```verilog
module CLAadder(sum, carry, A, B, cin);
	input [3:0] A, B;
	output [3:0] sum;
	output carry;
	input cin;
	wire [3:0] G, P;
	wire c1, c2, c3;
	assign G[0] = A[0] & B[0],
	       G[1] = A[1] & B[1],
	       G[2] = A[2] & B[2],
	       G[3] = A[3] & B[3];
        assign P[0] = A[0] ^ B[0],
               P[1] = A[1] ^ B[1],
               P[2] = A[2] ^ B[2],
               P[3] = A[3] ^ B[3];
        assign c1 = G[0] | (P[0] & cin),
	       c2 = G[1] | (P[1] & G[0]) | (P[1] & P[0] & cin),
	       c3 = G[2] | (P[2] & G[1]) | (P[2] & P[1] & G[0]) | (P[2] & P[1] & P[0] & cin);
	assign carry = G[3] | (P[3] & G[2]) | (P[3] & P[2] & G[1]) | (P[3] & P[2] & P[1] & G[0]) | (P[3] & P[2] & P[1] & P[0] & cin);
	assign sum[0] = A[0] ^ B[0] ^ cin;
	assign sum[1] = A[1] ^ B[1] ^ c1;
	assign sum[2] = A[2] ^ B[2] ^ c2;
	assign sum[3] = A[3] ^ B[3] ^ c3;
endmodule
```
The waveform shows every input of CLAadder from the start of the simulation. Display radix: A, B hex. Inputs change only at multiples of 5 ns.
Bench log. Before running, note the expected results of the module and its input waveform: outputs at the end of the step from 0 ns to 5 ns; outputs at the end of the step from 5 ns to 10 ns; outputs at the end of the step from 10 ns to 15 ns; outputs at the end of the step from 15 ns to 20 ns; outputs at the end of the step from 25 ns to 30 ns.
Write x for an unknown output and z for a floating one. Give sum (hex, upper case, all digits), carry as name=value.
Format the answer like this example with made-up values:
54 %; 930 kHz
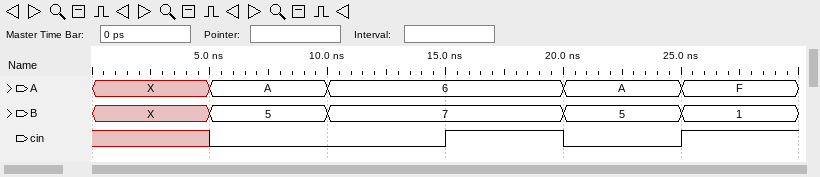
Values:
sum=x, carry=x; sum=F, carry=0; sum=D, carry=0; sum=E, carry=0; sum=1, carry=1
